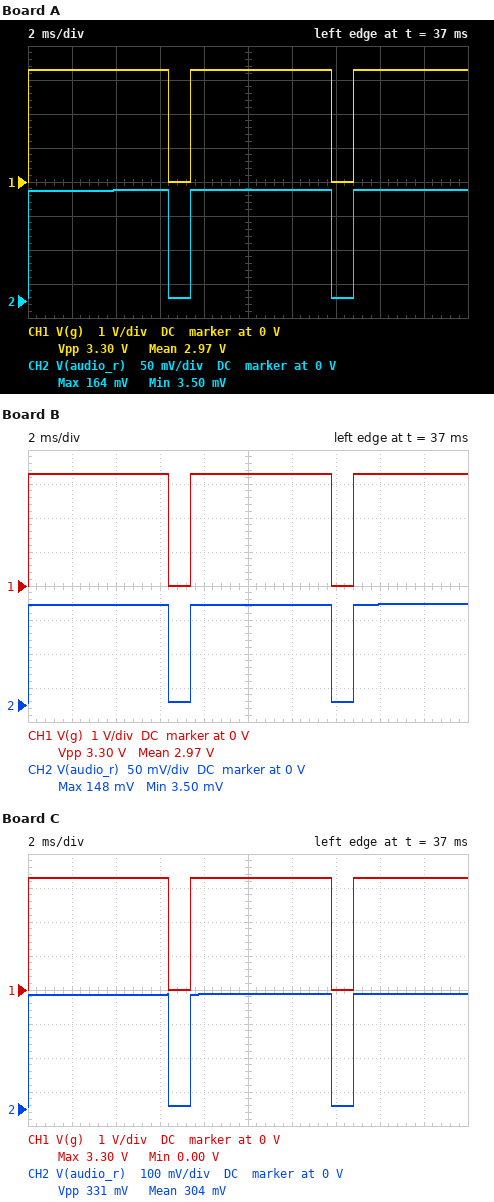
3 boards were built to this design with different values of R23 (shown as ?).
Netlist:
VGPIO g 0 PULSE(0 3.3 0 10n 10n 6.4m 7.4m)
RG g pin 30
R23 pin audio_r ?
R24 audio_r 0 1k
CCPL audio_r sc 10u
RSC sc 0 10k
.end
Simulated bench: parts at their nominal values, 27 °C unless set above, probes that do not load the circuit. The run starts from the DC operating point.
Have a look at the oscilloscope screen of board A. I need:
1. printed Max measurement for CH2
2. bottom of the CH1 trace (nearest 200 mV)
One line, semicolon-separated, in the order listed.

164 mV; 0 V
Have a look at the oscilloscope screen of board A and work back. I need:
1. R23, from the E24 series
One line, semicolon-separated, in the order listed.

18 kΩ
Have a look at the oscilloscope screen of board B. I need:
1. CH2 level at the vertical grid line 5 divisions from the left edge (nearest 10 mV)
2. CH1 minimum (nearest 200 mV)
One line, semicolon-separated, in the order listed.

150 mV; 0 V
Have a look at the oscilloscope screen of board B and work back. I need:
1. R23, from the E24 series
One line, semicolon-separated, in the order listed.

20 kΩ
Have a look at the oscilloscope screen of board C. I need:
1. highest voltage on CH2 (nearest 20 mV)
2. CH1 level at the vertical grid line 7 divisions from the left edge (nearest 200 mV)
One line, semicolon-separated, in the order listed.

340 mV; 0 V
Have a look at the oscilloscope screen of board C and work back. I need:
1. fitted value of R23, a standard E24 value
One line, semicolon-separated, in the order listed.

8.2 kΩ
